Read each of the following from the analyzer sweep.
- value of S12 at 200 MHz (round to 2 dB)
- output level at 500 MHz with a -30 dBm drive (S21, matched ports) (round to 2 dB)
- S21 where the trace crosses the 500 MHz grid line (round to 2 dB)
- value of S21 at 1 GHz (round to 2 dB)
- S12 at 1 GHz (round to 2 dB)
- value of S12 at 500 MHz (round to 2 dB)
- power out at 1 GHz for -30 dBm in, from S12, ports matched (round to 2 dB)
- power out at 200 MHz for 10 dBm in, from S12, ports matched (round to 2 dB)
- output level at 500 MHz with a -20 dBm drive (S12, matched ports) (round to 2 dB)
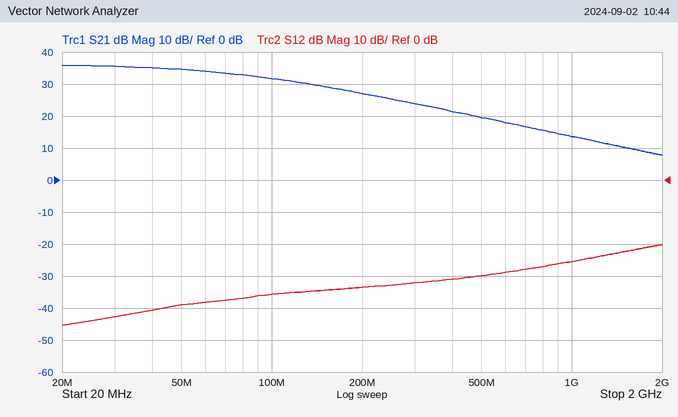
-34 dB
-10 dBm
20 dB
14 dB
-26 dB
-30 dB
-56 dBm
-24 dBm
-50 dBm
